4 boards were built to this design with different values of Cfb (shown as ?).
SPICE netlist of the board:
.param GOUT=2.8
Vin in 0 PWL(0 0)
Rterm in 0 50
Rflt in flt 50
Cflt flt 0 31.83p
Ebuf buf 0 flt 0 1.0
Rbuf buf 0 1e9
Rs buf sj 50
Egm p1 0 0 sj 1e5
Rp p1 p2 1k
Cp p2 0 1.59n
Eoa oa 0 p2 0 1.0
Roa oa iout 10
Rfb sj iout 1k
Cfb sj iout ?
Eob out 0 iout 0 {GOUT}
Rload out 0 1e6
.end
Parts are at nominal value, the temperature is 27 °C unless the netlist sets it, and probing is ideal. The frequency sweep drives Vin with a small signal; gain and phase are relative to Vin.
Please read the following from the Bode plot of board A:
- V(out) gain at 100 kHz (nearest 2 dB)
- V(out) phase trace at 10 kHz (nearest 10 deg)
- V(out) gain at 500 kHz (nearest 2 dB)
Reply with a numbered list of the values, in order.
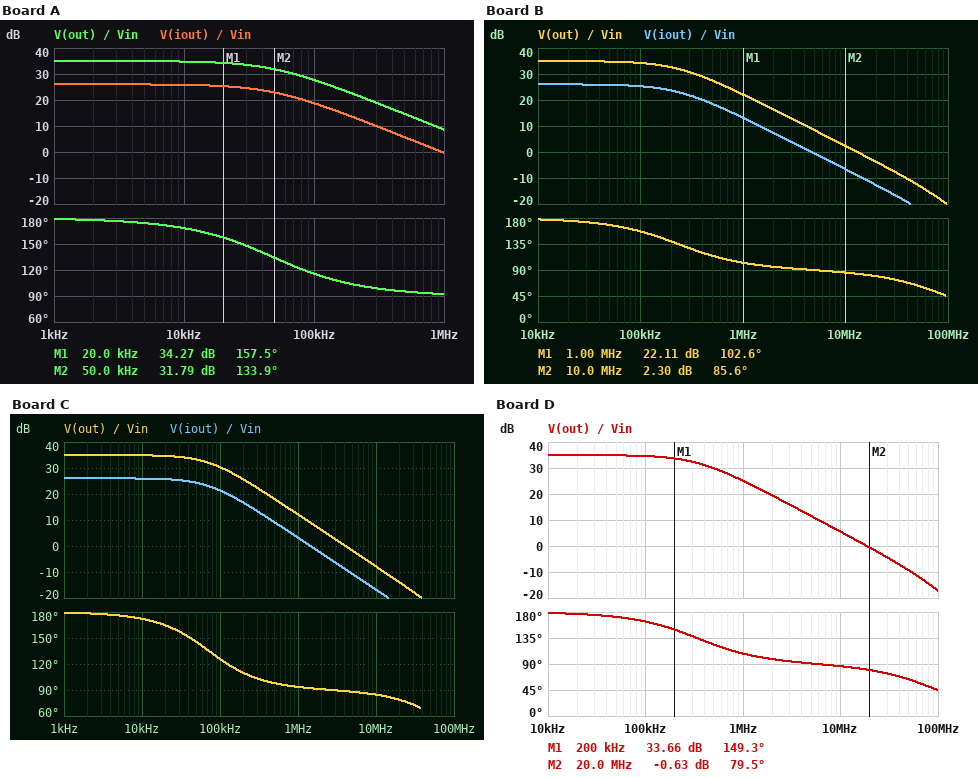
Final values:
1. 28 dB
2. 170 deg
3. 14 dB
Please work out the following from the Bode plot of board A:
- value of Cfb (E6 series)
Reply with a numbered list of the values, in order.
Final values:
1. 3.3 nF
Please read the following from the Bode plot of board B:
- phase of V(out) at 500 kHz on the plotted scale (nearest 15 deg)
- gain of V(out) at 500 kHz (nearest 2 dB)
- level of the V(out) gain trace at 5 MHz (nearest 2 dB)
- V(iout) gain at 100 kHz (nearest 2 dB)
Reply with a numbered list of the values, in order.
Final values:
1. 120 deg
2. 28 dB
3. 8 dB
4. 26 dB
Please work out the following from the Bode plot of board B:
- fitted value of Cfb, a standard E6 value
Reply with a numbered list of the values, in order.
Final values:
1. 680 pF
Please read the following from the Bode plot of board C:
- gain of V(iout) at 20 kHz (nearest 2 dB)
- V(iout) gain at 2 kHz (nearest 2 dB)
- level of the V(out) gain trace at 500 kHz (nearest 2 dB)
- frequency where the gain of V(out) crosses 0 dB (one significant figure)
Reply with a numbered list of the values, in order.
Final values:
1. 26 dB
2. 26 dB
3. 18 dB
4. 4 MHz
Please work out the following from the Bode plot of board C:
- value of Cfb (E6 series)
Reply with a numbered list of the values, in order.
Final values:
1. 2.2 nF
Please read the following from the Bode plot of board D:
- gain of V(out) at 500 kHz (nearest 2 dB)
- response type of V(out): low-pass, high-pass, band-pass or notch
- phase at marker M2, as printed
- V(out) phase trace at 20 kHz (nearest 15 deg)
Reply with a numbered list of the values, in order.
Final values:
1. 30 dB
2. low-pass
3. 79.5 deg
4. 180 deg
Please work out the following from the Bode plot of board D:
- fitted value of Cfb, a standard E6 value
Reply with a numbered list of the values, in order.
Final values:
1. 470 pF
